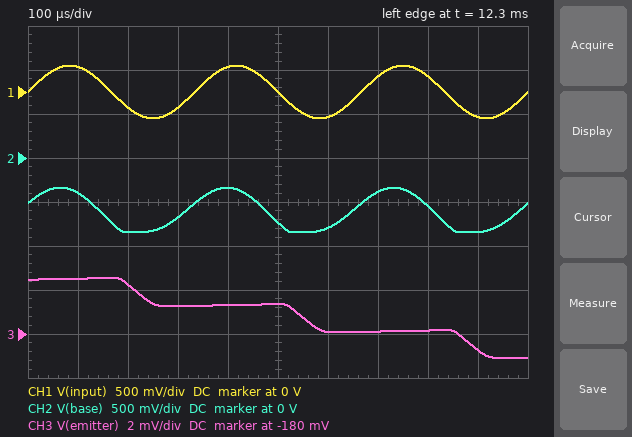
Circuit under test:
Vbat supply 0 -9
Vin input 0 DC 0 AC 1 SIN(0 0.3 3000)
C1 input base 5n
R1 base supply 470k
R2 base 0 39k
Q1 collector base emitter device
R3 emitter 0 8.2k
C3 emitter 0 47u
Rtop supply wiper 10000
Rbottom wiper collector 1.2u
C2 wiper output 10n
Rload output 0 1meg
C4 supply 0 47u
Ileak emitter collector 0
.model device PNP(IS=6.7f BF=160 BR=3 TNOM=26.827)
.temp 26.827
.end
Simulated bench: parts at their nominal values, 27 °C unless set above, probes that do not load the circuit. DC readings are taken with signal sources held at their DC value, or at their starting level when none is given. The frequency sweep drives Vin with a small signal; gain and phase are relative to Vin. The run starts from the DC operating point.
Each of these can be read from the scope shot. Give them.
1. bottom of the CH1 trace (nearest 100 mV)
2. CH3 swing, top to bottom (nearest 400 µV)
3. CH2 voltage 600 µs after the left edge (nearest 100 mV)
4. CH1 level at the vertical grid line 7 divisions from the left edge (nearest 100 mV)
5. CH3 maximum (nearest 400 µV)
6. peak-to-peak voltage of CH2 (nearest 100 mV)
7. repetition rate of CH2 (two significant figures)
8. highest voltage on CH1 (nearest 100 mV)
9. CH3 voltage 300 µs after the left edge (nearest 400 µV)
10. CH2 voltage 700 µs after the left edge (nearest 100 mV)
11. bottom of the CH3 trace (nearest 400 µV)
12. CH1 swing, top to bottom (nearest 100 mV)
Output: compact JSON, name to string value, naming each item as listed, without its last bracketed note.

{"bottom of the CH1 trace": "-300 mV", "CH3 swing, top to bottom": "3.6 mV", "CH2 voltage 600 µs after the left edge": "-800 mV", "CH1 level at the vertical grid line 7 divisions from the left edge": "200 mV", "CH3 maximum": "-177.6 mV", "peak-to-peak voltage of CH2": "500 mV", "repetition rate of CH2": "3.0 kHz", "highest voltage on CH1": "300 mV", "CH3 voltage 300 µs after the left edge": "-178.8 mV", "CH2 voltage 700 µs after the left edge": "-400 mV", "bottom of the CH3 trace": "-181.2 mV", "CH1 swing, top to bottom": "600 mV"}
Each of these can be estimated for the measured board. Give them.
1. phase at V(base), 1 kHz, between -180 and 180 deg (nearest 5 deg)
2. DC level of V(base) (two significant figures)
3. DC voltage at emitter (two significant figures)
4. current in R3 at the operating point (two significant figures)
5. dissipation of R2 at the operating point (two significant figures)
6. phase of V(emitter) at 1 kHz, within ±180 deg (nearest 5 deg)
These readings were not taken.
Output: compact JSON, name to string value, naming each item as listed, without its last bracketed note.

{"phase at V(base), 1 kHz, between -180 and 180 deg": "45 deg", "DC level of V(base)": "-690 mV", "DC voltage at emitter": "-130 mV", "current in R3 at the operating point": "16 µA", "dissipation of R2 at the operating point": "12 µW", "phase of V(emitter) at 1 kHz, within ±180 deg": "-45 deg"}
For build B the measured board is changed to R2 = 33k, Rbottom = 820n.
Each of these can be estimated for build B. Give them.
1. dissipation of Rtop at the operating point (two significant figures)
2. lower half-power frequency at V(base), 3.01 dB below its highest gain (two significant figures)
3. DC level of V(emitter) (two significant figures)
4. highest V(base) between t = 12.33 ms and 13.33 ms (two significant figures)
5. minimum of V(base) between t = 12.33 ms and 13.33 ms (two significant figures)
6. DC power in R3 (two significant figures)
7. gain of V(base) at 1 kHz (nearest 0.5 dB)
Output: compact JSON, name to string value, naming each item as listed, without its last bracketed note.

{"dissipation of Rtop at the operating point": "430 nW", "lower half-power frequency at V(base), 3.01 dB below its highest gain": "1.1 kHz", "DC level of V(emitter)": "-54 mV", "highest V(base) between t = 12.33 ms and 13.33 ms": "-260 mV", "minimum of V(base) between t = 12.33 ms and 13.33 ms": "-770 mV", "DC power in R3": "360 nW", "gain of V(base) at 1 kHz": "-3.5 dB"}
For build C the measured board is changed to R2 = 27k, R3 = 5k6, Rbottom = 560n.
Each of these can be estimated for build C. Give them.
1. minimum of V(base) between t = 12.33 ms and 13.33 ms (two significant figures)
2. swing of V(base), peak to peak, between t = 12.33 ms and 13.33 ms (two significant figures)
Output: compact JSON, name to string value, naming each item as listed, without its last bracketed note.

{"minimum of V(base) between t = 12.33 ms and 13.33 ms": "-710 mV", "swing of V(base), peak to peak, between t = 12.33 ms and 13.33 ms": "520 mV"}
